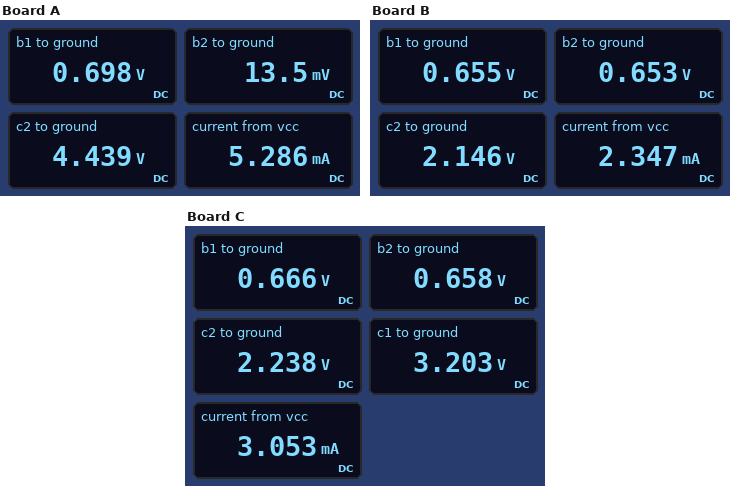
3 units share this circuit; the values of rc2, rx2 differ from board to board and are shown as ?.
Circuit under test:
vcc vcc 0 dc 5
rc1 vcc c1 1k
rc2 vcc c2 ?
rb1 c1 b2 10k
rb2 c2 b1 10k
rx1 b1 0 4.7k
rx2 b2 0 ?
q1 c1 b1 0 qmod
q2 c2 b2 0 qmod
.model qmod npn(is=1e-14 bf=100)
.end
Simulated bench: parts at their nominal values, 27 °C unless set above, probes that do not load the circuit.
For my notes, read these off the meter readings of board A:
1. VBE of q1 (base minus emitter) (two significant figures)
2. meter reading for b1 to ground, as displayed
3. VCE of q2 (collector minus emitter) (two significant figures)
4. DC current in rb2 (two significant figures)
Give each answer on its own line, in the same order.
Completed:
700 mV
0.698 V
4.4 V
370 µA
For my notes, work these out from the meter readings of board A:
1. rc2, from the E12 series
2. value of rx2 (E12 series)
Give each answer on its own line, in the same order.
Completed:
1.5 kΩ
1.8 kΩ
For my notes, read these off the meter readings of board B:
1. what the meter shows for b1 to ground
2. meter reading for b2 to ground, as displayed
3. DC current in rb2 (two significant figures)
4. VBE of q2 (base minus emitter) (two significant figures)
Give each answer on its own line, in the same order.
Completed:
0.655 V
0.653 V
150 µA
650 mV
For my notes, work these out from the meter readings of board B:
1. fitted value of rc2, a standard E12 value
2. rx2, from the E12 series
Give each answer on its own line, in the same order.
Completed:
2.7 kΩ
2.2 kΩ
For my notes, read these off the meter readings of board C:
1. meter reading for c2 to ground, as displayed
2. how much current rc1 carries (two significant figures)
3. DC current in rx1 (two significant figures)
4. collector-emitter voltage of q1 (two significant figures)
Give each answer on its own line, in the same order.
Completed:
2.238 V
1.8 mA
140 µA
3.2 V
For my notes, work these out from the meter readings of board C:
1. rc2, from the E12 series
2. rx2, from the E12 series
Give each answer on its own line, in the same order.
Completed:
2.2 kΩ
2.7 kΩ
